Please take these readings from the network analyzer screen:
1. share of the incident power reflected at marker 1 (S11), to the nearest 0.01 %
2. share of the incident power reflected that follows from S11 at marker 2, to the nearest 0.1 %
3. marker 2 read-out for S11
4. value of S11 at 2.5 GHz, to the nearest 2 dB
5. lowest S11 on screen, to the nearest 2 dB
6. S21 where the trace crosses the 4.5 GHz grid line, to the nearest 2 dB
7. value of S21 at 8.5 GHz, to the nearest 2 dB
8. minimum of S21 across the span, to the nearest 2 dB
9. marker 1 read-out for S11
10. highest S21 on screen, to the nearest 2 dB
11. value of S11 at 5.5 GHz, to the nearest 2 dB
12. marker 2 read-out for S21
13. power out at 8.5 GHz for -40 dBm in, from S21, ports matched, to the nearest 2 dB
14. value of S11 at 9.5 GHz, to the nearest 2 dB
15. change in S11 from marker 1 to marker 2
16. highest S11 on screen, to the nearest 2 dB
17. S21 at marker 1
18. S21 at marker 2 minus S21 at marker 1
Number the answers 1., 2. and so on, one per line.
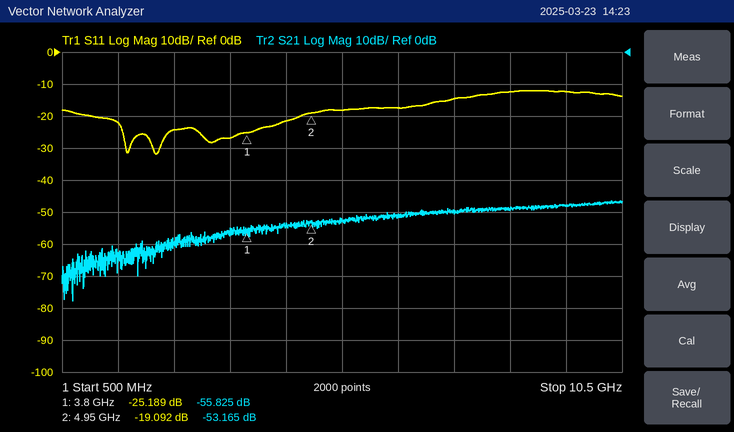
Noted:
1. 0.30 %
2. 1.2 %
3. -19.092 dB
4. -24 dB
5. -32 dB
6. -54 dB
7. -50 dB
8. -78 dB
9. -25.189 dB
10. -46 dB
11. -18 dB
12. -53.165 dB
13. -90 dBm
14. -12 dB
15. 6.097 dB
16. -12 dB
17. -55.825 dB
18. 2.660 dB
